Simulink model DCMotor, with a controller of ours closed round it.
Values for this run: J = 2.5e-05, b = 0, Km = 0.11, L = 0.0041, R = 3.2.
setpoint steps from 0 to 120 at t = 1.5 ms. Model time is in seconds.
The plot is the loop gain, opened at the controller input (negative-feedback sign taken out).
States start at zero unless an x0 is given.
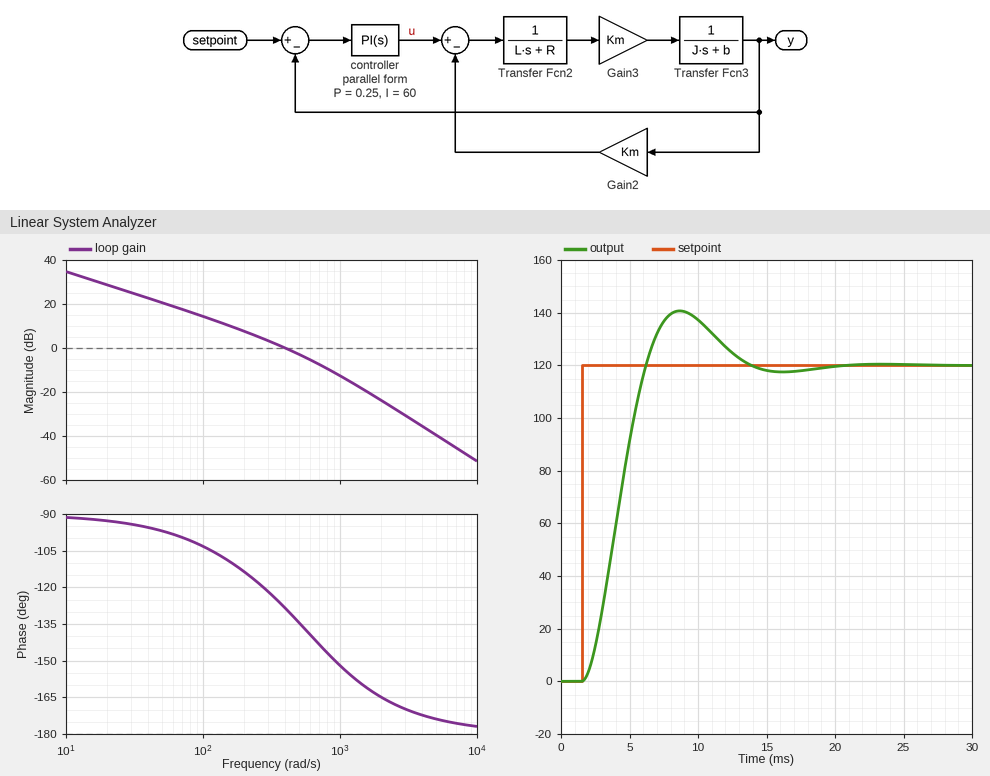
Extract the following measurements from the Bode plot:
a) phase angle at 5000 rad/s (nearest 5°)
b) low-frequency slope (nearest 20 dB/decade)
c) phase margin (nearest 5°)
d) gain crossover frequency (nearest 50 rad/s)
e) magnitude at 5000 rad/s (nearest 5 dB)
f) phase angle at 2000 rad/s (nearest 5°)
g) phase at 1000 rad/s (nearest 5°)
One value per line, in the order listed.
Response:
-175°
-20 dB/decade
50°
400 rad/s
-40 dB
-165°
-150°
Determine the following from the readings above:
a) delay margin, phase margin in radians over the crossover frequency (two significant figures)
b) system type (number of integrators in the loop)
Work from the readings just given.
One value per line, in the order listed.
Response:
0.0022 s
1
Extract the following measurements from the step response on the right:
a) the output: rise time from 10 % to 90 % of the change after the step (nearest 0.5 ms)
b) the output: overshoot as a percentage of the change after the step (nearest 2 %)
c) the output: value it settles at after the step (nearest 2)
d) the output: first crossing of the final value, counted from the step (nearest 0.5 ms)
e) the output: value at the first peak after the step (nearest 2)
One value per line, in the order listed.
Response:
3.0 ms
18 %
120
4.5 ms
140
